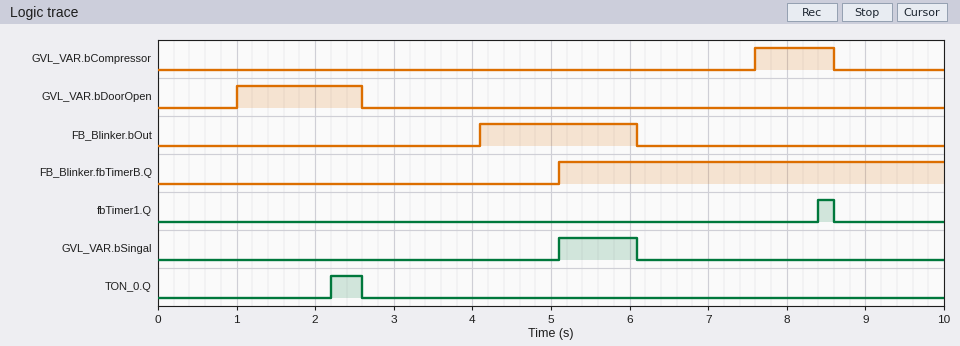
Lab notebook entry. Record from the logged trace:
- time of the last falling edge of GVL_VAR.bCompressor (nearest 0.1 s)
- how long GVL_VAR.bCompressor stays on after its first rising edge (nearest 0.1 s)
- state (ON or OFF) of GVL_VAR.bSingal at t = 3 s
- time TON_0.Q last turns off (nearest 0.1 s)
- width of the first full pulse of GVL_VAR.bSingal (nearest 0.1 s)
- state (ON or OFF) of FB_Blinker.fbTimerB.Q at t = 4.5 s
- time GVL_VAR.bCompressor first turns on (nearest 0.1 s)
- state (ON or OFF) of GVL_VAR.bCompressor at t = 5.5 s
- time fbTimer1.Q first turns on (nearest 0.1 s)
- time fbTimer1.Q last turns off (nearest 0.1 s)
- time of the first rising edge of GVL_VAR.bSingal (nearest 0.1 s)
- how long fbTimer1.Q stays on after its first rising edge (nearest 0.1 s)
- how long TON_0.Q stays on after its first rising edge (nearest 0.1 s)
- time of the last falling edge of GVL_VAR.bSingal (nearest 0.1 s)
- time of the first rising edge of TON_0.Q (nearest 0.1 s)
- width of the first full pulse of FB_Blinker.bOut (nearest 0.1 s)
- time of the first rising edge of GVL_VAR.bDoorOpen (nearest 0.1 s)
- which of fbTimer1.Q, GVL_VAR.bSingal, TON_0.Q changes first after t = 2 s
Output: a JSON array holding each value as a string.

["8.6 s", "1.0 s", "OFF", "2.6 s", "1.0 s", "OFF", "7.6 s", "OFF", "8.4 s", "8.6 s", "5.1 s", "0.2 s", "0.4 s", "6.1 s", "2.2 s", "2.0 s", "1.0 s", "TON_0.Q"]
